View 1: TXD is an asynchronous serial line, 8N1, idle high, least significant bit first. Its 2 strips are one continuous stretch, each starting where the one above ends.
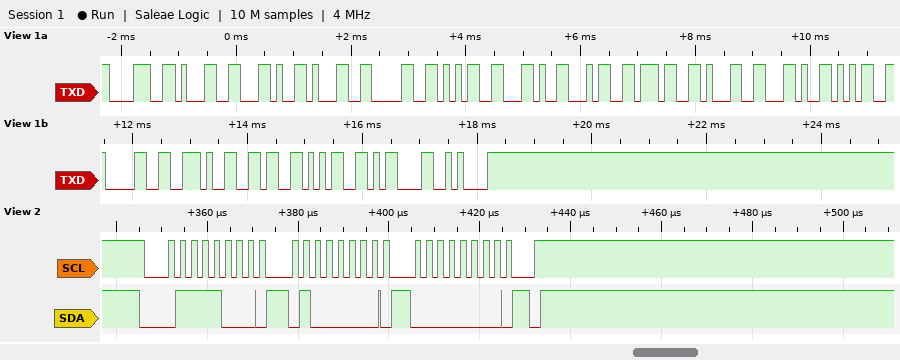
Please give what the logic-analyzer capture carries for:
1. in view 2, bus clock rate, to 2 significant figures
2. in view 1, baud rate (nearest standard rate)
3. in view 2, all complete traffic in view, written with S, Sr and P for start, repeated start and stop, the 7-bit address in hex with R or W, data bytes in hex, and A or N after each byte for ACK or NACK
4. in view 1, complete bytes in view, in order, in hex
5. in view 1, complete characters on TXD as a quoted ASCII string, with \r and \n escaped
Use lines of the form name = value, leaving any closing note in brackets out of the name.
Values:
in view 2, bus clock rate, to 2 significant figures = 400 kHz
in view 1, baud rate = 9600 baud
in view 2, all complete traffic in view, written with S, Sr and P for start, repeated start and stop, the 7-bit address in hex with R or W, data bytes in hex, and A or N after each byte for ACK or NACK = S 3CW A 40 A 00 A P
in view 1, complete bytes in view, in order, in hex = 0x38 0x31 0x2C 0x31 0x30 0x35 0x2C 0x34 0x37 0x31 0x2C 0x35 0x30 0x2E 0x36 0x35 0x0D 0x0A
in view 1, complete characters on TXD as a quoted ASCII string, with \r and \n escaped = "81,105,471,50.65\r\n"
